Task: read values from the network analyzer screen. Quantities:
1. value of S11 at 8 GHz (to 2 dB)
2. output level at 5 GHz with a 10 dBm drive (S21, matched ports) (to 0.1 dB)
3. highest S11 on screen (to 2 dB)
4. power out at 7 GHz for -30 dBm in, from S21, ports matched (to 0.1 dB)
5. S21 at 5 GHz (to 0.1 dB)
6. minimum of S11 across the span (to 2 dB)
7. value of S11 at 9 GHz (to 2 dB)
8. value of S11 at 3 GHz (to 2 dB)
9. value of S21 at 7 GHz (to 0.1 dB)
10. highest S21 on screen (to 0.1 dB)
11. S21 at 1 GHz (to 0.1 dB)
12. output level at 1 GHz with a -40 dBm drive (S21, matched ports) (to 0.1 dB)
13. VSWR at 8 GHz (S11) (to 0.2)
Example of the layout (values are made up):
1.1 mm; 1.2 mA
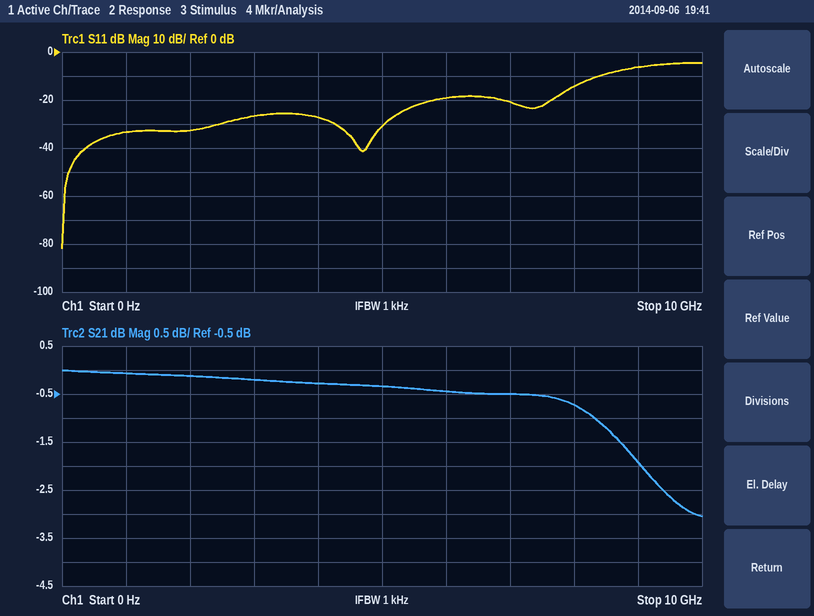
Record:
-14 dB; 9.7 dBm; -4 dB; -30.5 dBm; -0.3 dB; -82 dB; -6 dB; -26 dB; -0.5 dB; 0.0 dB; -0.1 dB; -40.1 dBm; 1.4
